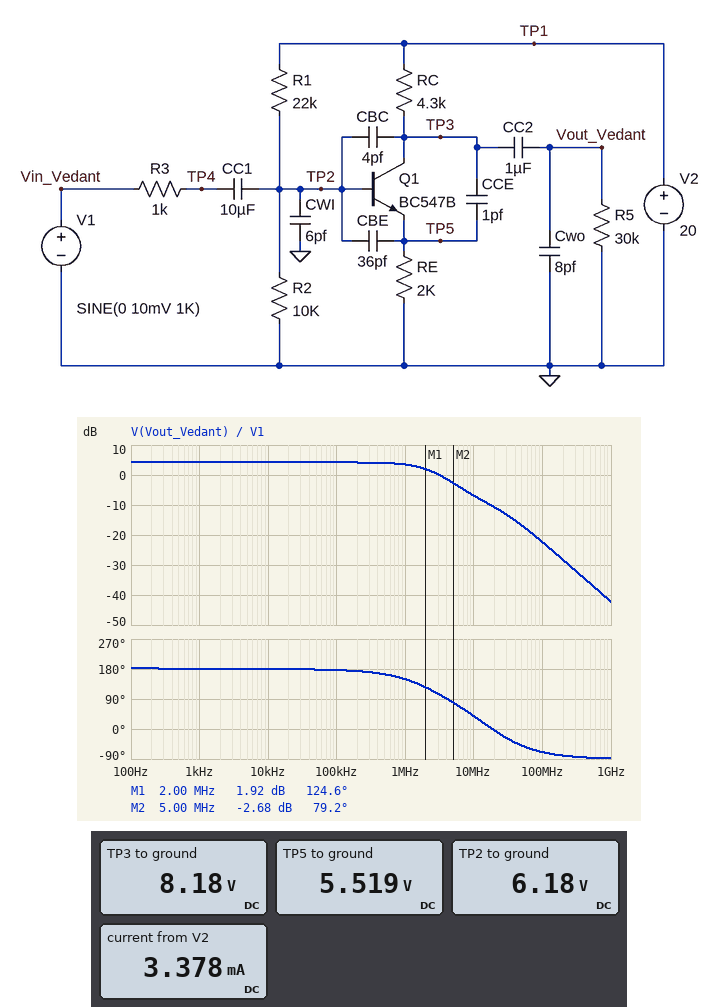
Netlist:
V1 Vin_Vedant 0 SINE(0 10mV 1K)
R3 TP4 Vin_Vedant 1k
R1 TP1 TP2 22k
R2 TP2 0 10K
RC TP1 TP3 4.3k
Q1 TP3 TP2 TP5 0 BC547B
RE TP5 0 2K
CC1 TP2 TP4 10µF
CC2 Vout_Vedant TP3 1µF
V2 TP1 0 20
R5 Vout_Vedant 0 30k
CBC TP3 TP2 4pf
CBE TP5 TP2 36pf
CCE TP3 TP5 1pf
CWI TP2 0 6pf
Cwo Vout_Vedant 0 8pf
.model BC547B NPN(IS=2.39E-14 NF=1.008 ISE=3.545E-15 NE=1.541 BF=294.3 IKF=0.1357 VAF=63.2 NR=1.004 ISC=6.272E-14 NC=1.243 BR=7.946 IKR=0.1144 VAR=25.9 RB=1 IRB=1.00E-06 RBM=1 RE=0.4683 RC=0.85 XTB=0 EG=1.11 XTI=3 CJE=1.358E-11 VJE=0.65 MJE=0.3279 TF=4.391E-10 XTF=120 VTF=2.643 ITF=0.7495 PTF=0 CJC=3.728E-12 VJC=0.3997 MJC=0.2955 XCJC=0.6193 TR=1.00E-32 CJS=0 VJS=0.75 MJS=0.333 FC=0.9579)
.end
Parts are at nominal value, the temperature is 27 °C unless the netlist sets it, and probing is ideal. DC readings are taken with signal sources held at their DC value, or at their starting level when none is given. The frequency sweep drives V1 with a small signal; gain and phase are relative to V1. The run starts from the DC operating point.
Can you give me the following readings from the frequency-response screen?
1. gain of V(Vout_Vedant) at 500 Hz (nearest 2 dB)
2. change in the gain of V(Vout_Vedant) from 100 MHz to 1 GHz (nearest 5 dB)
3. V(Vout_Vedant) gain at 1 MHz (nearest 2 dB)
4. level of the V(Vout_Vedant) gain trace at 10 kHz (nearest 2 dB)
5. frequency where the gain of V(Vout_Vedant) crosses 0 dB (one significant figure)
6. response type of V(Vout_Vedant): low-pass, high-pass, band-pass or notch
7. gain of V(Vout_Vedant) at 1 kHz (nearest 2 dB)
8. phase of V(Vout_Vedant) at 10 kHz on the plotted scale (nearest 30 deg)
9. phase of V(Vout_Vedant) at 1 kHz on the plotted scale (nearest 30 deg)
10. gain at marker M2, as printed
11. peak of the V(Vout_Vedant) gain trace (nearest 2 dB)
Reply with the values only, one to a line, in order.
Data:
4 dB
-20 dB
4 dB
4 dB
3 MHz
low-pass
4 dB
180 deg
180 deg
-2.68 dB
4 dB
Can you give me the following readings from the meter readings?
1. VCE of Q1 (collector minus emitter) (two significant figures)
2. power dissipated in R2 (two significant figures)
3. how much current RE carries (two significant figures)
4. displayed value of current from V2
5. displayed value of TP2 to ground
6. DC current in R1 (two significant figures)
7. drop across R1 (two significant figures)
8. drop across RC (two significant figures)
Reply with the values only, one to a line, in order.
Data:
2.7 V
3.8 mW
2.8 mA
3.378 mA
6.18 V
630 µA
14 V
12 V
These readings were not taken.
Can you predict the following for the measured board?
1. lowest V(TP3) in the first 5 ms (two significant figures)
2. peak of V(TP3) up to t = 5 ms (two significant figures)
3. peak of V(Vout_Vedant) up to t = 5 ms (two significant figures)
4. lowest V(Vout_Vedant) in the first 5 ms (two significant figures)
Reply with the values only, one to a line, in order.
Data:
8.2 V
8.2 V
16 mV
-16 mV
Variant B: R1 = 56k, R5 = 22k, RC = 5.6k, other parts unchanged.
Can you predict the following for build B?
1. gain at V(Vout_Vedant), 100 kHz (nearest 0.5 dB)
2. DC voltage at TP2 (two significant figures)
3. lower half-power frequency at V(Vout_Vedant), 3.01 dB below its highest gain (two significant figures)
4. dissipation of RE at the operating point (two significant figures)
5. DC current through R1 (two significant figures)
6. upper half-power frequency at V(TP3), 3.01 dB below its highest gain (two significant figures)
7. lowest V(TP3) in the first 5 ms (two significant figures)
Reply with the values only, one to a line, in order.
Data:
6.0 dB
3.0 V
6.2 Hz
2.8 mW
300 µA
1.8 MHz
13 V
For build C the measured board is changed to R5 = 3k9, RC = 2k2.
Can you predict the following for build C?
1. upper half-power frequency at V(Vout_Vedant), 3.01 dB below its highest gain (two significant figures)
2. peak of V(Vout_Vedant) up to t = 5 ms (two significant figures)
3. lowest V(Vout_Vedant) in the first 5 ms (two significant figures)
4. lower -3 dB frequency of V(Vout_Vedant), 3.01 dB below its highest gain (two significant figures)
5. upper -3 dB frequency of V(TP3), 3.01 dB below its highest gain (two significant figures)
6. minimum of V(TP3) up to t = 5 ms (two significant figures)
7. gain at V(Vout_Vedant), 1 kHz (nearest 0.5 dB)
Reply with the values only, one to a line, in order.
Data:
7.1 MHz
6.2 mV
-6.0 mV
26 Hz
100 Hz
14 V
-4.5 dB
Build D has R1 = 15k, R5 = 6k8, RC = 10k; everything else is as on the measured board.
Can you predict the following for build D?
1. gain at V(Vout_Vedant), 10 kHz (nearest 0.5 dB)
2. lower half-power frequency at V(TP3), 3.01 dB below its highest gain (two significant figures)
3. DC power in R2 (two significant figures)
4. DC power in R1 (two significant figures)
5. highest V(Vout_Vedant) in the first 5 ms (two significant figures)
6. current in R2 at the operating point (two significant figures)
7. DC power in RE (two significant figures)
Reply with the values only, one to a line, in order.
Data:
-6.0 dB
6.1 Hz
2.4 mW
15 mW
5.0 mV
490 µA
8.8 mW
